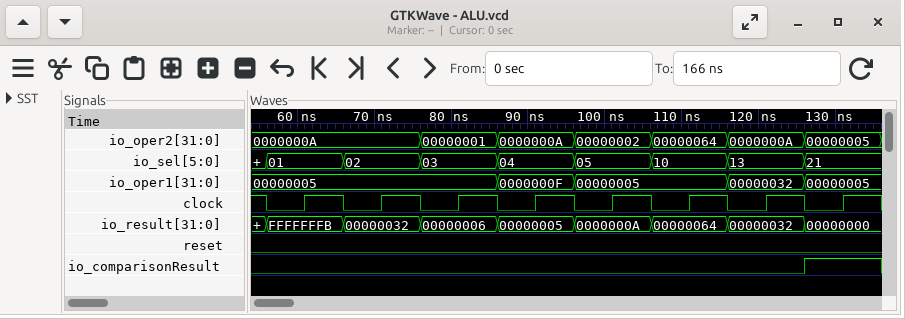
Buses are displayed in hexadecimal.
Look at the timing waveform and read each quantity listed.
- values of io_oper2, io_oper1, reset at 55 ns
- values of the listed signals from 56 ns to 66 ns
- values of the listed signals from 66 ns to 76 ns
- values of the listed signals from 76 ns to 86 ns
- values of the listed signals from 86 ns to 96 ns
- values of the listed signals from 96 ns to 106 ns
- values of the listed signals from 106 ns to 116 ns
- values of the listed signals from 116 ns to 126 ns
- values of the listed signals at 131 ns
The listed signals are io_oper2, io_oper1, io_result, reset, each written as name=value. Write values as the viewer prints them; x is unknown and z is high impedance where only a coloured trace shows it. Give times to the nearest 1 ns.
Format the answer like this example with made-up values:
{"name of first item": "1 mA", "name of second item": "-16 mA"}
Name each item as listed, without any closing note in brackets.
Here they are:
{"values of io_oper2, io_oper1, reset at 55 ns": "io_oper2=0000000A, io_oper1=00000005, reset=0", "values of the listed signals from 56 ns to 66 ns": "io_oper2=0000000A, io_oper1=00000005, io_result=FFFFFFFB, reset=0", "values of the listed signals from 66 ns to 76 ns": "io_oper2=0000000A, io_oper1=00000005, io_result=00000032, reset=0", "values of the listed signals from 76 ns to 86 ns": "io_oper2=00000001, io_oper1=00000005, io_result=00000006, reset=0", "values of the listed signals from 86 ns to 96 ns": "io_oper2=0000000A, io_oper1=0000000F, io_result=00000005, reset=0", "values of the listed signals from 96 ns to 106 ns": "io_oper2=00000002, io_oper1=00000005, io_result=0000000A, reset=0", "values of the listed signals from 106 ns to 116 ns": "io_oper2=00000064, io_oper1=00000005, io_result=00000064, reset=0", "values of the listed signals from 116 ns to 126 ns": "io_oper2=0000000A, io_oper1=00000032, io_result=00000032, reset=0", "values of the listed signals at 131 ns": "io_oper2=00000005, io_oper1=00000005, io_result=00000000, reset=0"}
